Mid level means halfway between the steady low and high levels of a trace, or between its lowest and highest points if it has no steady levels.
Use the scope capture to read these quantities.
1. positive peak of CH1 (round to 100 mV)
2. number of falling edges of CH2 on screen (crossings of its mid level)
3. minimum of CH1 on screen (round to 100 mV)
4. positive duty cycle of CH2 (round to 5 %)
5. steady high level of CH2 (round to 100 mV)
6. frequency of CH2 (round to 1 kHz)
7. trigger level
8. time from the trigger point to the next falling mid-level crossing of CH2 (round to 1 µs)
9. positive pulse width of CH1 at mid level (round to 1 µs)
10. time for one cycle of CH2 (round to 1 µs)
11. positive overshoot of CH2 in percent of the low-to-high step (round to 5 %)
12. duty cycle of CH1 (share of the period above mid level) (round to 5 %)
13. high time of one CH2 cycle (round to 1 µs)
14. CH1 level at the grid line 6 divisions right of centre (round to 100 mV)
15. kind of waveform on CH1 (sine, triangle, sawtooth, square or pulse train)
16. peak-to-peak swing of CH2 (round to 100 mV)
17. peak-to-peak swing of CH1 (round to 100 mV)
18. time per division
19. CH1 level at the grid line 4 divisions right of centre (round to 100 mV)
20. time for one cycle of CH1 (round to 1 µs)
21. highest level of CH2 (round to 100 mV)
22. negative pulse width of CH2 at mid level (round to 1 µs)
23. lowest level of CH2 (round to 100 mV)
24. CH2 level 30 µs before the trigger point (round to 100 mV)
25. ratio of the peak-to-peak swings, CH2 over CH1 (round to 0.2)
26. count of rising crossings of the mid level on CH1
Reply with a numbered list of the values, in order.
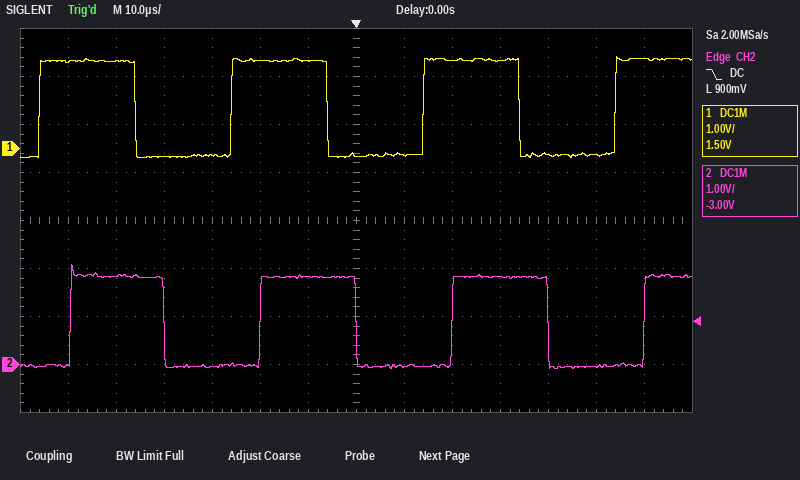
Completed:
1. 1.9 V
2. 3
3. -200 mV
4. 50 %
5. 1.8 V
6. 25 kHz
7. 900 mV
8. 40 µs
9. 20 µs
10. 40 µs
11. 15 %
12. 50 %
13. 20 µs
14. 1.9 V
15. square
16. 2.2 V
17. 2.1 V
18. 10 µs
19. -100 mV
20. 40 µs
21. 2.1 V
22. 20 µs
23. -100 mV
24. 0.0 V
25. 1.0
26. 4
